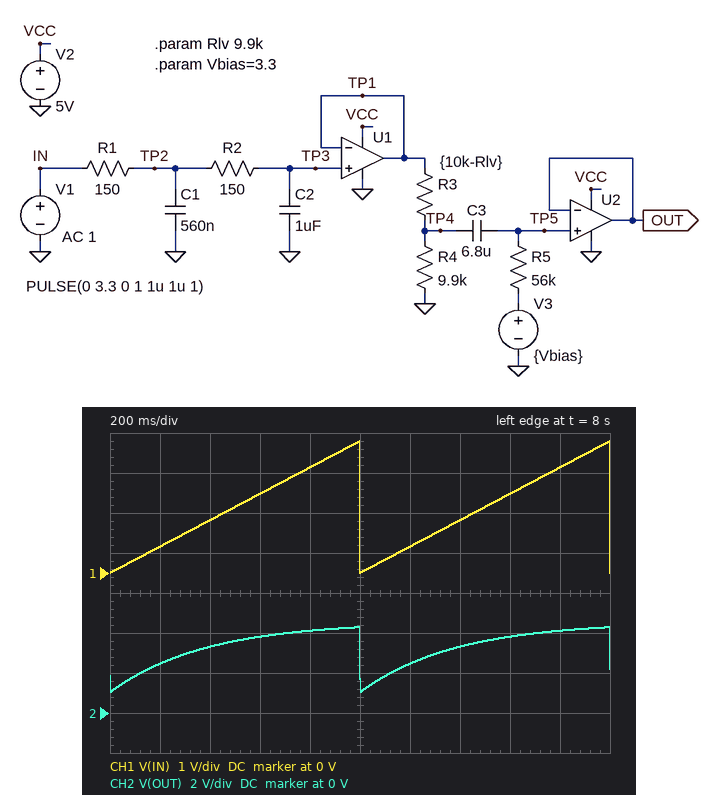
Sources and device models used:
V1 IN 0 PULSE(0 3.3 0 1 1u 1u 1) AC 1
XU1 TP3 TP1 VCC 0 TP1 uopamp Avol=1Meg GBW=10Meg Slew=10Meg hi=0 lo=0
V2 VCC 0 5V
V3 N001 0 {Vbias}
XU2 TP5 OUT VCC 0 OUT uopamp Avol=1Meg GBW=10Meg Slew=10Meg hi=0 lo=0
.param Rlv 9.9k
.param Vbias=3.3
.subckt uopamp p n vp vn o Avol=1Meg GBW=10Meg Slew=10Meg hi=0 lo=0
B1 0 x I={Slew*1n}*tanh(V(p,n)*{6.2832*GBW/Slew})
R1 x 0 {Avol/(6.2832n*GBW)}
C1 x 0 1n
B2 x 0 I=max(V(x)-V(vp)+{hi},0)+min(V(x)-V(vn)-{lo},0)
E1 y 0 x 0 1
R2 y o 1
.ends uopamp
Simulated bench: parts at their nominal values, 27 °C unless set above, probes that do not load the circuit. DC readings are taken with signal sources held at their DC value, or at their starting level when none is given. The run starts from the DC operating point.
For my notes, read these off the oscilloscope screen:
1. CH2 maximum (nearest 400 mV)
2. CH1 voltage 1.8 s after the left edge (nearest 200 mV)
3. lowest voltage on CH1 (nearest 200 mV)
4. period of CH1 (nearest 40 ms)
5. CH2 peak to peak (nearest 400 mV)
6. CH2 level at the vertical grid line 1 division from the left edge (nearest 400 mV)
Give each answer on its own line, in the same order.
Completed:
4.4 V
2.6 V
0 V
1.00 s
3.2 V
2.4 V
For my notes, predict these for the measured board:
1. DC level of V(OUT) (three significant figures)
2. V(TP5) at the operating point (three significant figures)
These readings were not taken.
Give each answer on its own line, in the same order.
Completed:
3.30 V
3.30 V
